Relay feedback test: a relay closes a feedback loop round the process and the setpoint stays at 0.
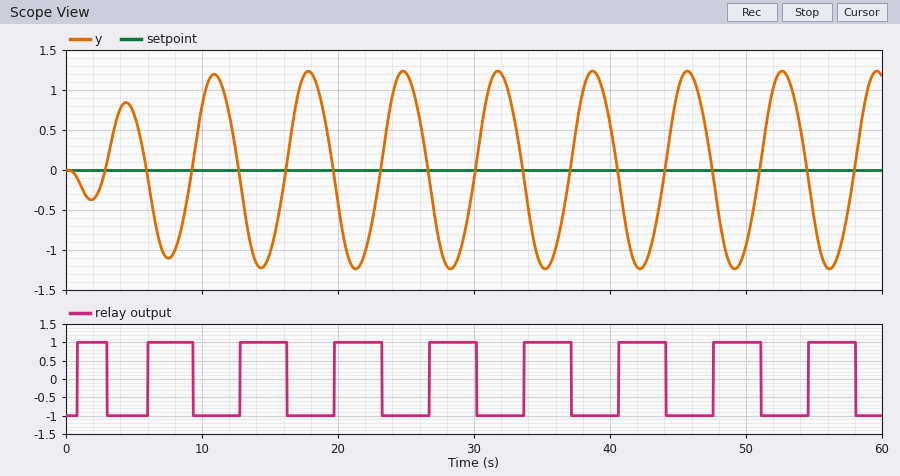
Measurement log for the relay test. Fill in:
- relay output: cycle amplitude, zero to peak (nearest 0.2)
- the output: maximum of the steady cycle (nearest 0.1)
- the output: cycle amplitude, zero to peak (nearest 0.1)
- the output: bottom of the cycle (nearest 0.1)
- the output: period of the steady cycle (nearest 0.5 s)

1.0
1.2
1.2
-1.2
7.0 s
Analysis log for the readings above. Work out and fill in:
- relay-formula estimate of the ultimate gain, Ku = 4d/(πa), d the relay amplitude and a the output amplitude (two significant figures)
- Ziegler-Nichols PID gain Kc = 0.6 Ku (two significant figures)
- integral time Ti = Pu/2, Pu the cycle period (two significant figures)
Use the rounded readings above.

1.1
0.66
3.5 s
